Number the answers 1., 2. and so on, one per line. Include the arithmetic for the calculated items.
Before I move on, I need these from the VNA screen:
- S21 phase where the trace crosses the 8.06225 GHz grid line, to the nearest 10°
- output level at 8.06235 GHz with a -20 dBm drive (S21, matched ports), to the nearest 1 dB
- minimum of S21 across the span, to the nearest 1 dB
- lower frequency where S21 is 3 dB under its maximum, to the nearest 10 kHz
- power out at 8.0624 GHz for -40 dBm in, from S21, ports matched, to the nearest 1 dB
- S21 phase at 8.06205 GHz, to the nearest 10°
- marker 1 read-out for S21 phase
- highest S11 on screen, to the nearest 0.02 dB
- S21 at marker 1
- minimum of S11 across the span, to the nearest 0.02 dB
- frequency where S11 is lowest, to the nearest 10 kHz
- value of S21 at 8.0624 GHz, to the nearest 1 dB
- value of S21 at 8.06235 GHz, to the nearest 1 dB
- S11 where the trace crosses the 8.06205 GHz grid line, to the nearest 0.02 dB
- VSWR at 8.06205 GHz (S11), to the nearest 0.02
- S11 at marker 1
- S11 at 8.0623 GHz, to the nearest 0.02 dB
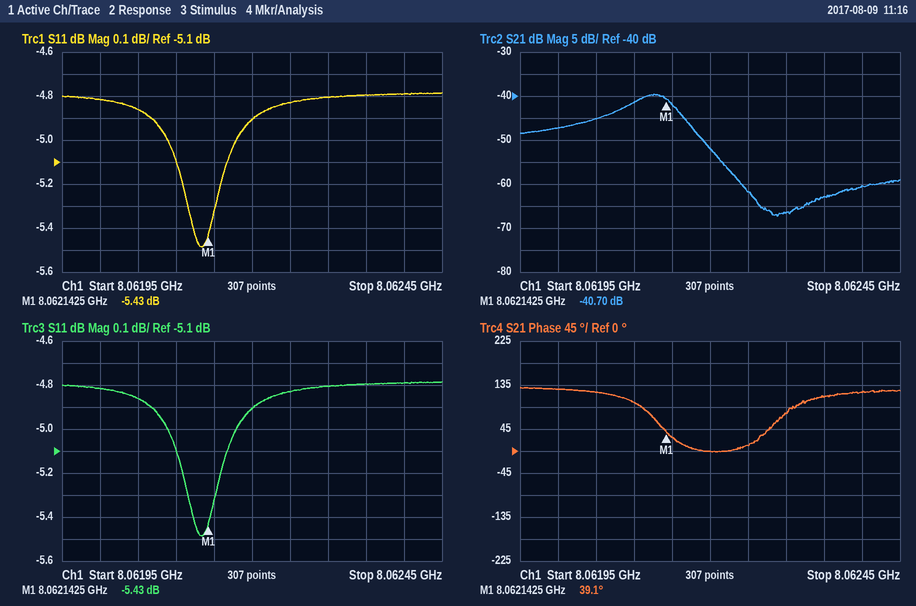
1. 10°
2. -20 dBm + (-63 dB) = -83 dBm
3. -67 dB
4. 8.06209 GHz
5. -40 dBm + (-60 dB) = -100 dBm
6. 120°
7. 39.1°
8. -4.78 dB
9. -40.70 dB
10. -5.48 dB
11. 8.06213 GHz
12. -60 dB
13. -63 dB
14. -4.86 dB
15. |Γ| = 10^(-4.86/20) = 0.5715; VSWR = (1 + 0.5715)/(1 − 0.5715) ≈ 3.67, so 3.66 to the nearest 0.02
16. -5.43 dB
17. -4.80 dB
